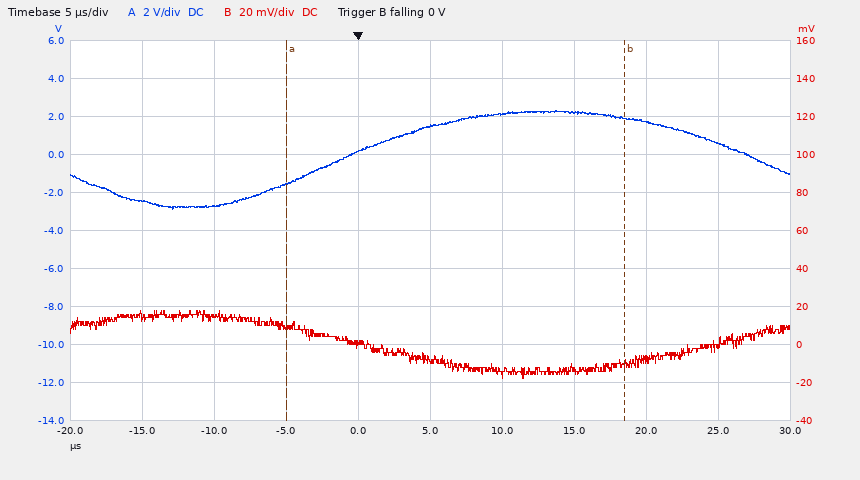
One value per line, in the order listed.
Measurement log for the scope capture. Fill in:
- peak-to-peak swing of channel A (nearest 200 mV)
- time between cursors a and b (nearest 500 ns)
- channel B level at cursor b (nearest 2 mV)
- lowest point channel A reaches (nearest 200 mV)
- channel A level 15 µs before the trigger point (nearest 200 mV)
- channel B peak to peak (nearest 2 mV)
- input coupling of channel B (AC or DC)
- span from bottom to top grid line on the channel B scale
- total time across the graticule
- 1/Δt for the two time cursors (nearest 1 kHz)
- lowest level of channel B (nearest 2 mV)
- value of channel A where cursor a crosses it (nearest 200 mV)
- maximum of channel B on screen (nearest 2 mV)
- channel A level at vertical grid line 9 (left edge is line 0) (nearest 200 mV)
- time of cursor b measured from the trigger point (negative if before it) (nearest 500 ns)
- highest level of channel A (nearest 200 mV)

5.2 V
23.5 µs
-10 mV
-2.8 V
-2.4 V
36 mV
DC
200 mV
50 µs
43 kHz
-18 mV
-1.6 V
18 mV
600 mV
+18.5 µs
2.4 V
